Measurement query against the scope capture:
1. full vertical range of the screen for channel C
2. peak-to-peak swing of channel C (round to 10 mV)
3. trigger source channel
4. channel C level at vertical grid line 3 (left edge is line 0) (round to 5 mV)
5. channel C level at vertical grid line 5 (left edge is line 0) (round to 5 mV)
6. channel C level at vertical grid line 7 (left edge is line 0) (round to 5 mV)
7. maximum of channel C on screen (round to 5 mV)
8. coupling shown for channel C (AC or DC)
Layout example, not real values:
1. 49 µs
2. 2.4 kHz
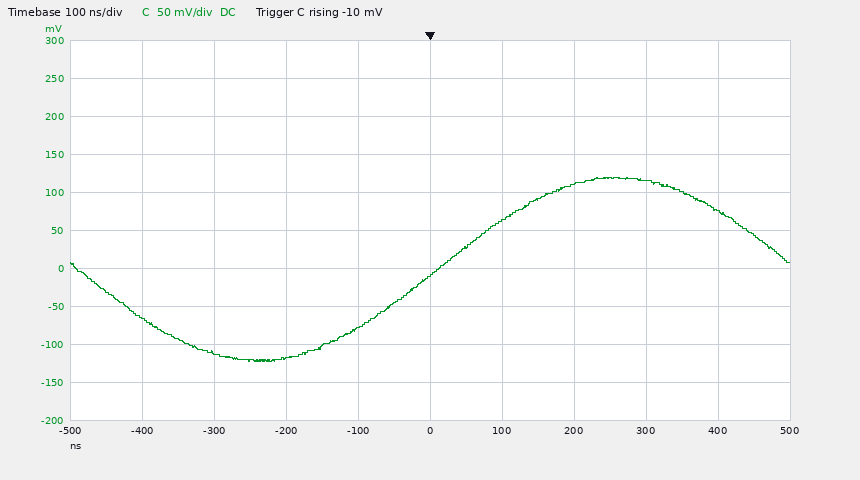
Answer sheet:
1. 500 mV
2. 240 mV
3. channel C
4. -120 mV
5. -10 mV
6. 110 mV
7. 120 mV
8. DC
